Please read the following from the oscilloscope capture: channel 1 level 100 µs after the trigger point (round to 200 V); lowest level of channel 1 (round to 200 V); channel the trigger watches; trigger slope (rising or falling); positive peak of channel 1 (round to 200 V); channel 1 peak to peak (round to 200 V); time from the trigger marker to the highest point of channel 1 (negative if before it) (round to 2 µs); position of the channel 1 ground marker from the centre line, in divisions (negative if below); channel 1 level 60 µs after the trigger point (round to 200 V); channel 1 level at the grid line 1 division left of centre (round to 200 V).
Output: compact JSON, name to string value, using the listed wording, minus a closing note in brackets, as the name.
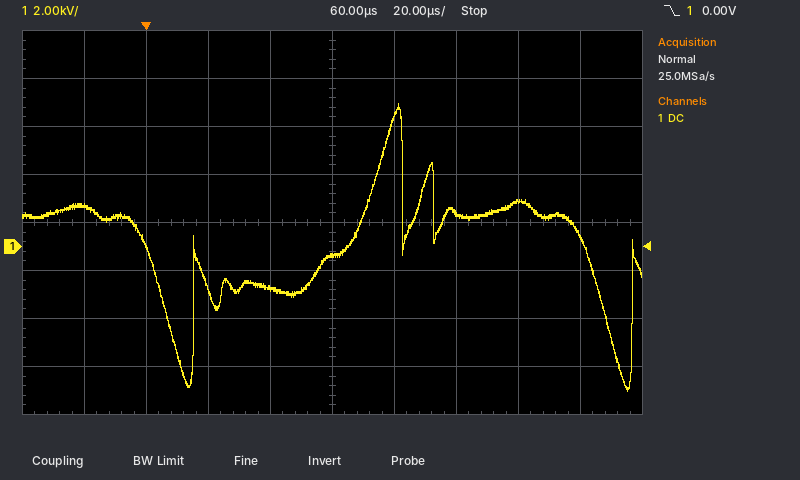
{"channel 1 level 100 µs after the trigger point": "1.4 kV", "lowest level of channel 1": "-6.0 kV", "channel the trigger watches": "channel 1", "trigger slope": "falling", "positive peak of channel 1": "6.0 kV", "channel 1 peak to peak": "12.0 kV", "time from the trigger marker to the highest point of channel 1 (negative if before it)": "+82 µs", "position of the channel 1 ground marker from the centre line, in divisions": "-0.5 div", "channel 1 level 60 µs after the trigger point": "-400 V", "channel 1 level at the grid line 1 division left of centre": "-1.8 kV"}
